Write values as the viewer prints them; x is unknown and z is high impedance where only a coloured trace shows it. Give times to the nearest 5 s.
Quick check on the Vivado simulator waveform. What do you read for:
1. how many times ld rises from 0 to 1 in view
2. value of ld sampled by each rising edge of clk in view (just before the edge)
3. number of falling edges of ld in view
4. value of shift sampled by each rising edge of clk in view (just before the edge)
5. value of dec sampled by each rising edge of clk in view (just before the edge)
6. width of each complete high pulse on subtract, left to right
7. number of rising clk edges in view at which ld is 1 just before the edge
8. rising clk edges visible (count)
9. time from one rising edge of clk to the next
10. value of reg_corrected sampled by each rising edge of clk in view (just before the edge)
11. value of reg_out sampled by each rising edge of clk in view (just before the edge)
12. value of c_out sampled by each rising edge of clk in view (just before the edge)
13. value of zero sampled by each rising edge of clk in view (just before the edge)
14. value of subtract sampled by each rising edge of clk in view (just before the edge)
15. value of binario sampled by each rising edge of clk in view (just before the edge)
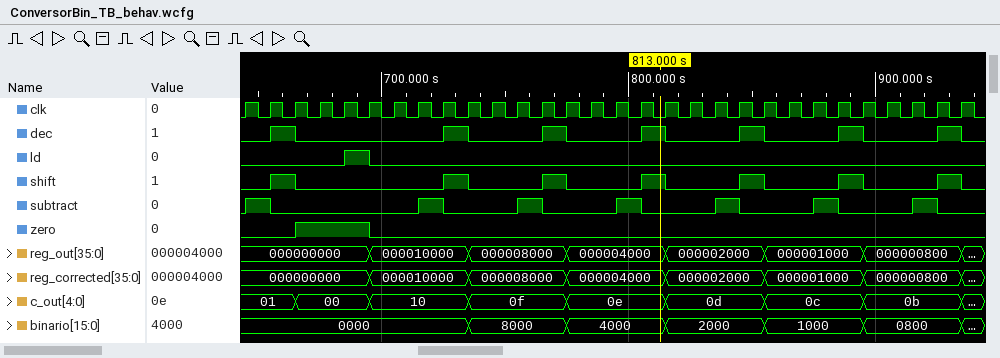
1
0 0 0 0 0 1 0 0 0 0 0 0 0 0 0 0 0 0 0 0 0 0 0 0 0 0 0 0 0 0
1
0 0 1 0 0 0 0 0 0 1 0 0 0 1 0 0 0 1 0 0 0 1 0 0 0 1 0 0 0 1
0 0 1 0 0 0 0 0 0 1 0 0 0 1 0 0 0 1 0 0 0 1 0 0 0 1 0 0 0 1
10 s, 10 s, 10 s, 10 s, 10 s, 10 s, 10 s
1
30
10 s
000000000, 000000000, 000000000, 000000000, 000000000, 000000000, 000010000, 000010000, 000010000, 000010000, 000008000, 000008000, 000008000, 000008000, 000004000, 000004000, 000004000, 000004000, 000002000, 000002000, 000002000, 000002000, 000001000, 000001000, 000001000, 000001000, 000000800, 000000800, 000000800, 000000800
000000000, 000000000, 000000000, 000000000, 000000000, 000000000, 000010000, 000010000, 000010000, 000010000, 000008000, 000008000, 000008000, 000008000, 000004000, 000004000, 000004000, 000004000, 000002000, 000002000, 000002000, 000002000, 000001000, 000001000, 000001000, 000001000, 000000800, 000000800, 000000800, 000000800
01, 01, 01, 00, 00, 00, 10, 10, 10, 10, 0f, 0f, 0f, 0f, 0e, 0e, 0e, 0e, 0d, 0d, 0d, 0d, 0c, 0c, 0c, 0c, 0b, 0b, 0b, 0b
0 0 0 1 1 1 0 0 0 0 0 0 0 0 0 0 0 0 0 0 0 0 0 0 0 0 0 0 0 0
0 1 0 0 0 0 0 0 1 0 0 0 1 0 0 0 1 0 0 0 1 0 0 0 1 0 0 0 1 0
0000, 0000, 0000, 0000, 0000, 0000, 0000, 0000, 0000, 0000, 8000, 8000, 8000, 8000, 4000, 4000, 4000, 4000, 2000, 2000, 2000, 2000, 1000, 1000, 1000, 1000, 0800, 0800, 0800, 0800
